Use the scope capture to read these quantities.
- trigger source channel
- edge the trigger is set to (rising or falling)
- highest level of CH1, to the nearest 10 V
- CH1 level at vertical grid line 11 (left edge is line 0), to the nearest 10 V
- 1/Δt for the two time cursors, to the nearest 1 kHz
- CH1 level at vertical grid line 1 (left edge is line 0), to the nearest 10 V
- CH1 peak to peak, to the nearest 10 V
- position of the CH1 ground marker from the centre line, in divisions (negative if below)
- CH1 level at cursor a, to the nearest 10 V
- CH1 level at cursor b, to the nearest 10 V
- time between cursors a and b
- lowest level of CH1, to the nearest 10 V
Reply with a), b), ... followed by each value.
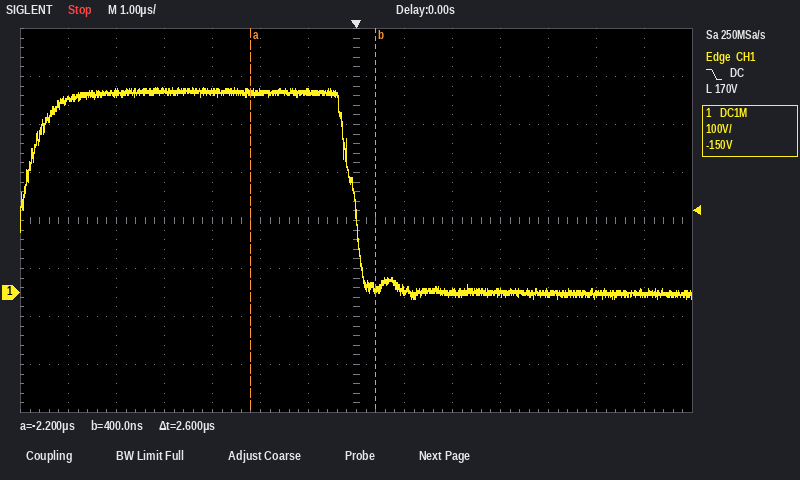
a) CH1
b) falling
c) 430 V
d) 0 V
e) 385 kHz
f) 400 V
g) 440 V
h) -1.5 div
i) 420 V
j) 10 V
k) 2.6 µs
l) -10 V
